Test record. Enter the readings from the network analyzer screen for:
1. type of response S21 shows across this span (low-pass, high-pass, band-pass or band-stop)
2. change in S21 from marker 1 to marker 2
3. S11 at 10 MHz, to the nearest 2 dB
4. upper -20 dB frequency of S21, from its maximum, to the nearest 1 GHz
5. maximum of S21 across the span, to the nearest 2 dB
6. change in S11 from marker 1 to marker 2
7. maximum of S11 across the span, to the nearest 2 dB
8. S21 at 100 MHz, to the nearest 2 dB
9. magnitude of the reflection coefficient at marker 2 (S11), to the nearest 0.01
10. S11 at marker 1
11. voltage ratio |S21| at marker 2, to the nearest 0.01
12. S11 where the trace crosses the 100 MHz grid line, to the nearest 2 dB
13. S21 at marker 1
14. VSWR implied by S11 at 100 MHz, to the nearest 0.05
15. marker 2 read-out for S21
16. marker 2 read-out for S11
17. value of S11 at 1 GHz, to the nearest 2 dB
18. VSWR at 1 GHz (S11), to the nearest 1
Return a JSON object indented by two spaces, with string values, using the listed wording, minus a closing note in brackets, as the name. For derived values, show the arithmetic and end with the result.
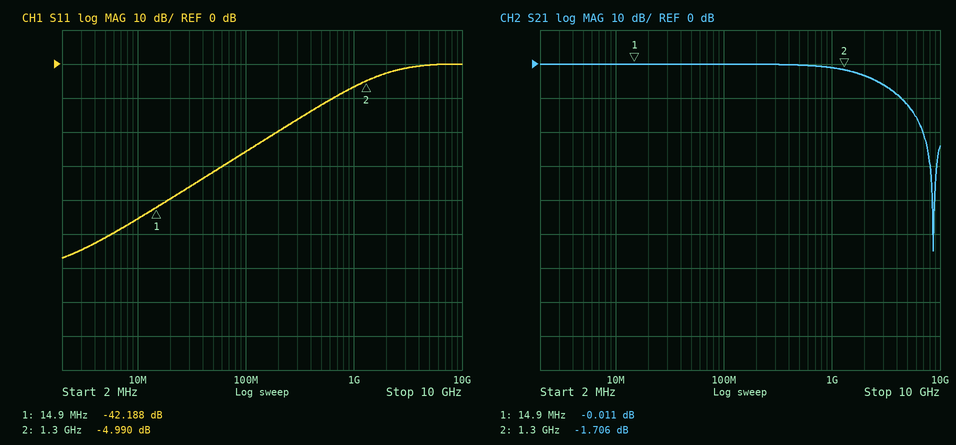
{
  "type of response S21 shows across this span": "low-pass",
  "change in S21 from marker 1 to marker 2": "-1.706 − (-0.011) = -1.695 dB",
  "S11 at 10 MHz, to the nearest 2 dB": "-46 dB",
  "upper -20 dB frequency of S21, from its maximum, to the nearest 1 GHz": "7 GHz",
  "maximum of S21 across the span, to the nearest 2 dB": "0 dB",
  "change in S11 from marker 1 to marker 2": "-4.99 − (-42.188) = 37.198 dB",
  "maximum of S11 across the span, to the nearest 2 dB": "0 dB",
  "S21 at 100 MHz, to the nearest 2 dB": "0 dB",
  "magnitude of the reflection coefficient at marker 2 (S11), to the nearest 0.01": "10^(-4.99/20) ≈ 0.56",
  "S11 at marker 1": "-42.188 dB",
  "voltage ratio |S21| at marker 2, to the nearest 0.01": "10^(-1.706/20) ≈ 0.82",
  "S11 where the trace crosses the 100 MHz grid line, to the nearest 2 dB": "-26 dB",
  "S21 at marker 1": "-0.011 dB",
  "VSWR implied by S11 at 100 MHz, to the nearest 0.05": "|Γ| = 10^(-26/20) = 0.0501; VSWR = (1 + 0.0501)/(1 − 0.0501) ≈ 1.11, so 1.10 to the nearest 0.05",
  "marker 2 read-out for S21": "-1.706 dB",
  "marker 2 read-out for S11": "-4.990 dB",
  "value of S11 at 1 GHz, to the nearest 2 dB": "-6 dB",
  "VSWR at 1 GHz (S11), to the nearest 1": "|Γ| = 10^(-6/20) = 0.5012; VSWR = (1 + 0.5012)/(1 − 0.5012) ≈ 3"
}
